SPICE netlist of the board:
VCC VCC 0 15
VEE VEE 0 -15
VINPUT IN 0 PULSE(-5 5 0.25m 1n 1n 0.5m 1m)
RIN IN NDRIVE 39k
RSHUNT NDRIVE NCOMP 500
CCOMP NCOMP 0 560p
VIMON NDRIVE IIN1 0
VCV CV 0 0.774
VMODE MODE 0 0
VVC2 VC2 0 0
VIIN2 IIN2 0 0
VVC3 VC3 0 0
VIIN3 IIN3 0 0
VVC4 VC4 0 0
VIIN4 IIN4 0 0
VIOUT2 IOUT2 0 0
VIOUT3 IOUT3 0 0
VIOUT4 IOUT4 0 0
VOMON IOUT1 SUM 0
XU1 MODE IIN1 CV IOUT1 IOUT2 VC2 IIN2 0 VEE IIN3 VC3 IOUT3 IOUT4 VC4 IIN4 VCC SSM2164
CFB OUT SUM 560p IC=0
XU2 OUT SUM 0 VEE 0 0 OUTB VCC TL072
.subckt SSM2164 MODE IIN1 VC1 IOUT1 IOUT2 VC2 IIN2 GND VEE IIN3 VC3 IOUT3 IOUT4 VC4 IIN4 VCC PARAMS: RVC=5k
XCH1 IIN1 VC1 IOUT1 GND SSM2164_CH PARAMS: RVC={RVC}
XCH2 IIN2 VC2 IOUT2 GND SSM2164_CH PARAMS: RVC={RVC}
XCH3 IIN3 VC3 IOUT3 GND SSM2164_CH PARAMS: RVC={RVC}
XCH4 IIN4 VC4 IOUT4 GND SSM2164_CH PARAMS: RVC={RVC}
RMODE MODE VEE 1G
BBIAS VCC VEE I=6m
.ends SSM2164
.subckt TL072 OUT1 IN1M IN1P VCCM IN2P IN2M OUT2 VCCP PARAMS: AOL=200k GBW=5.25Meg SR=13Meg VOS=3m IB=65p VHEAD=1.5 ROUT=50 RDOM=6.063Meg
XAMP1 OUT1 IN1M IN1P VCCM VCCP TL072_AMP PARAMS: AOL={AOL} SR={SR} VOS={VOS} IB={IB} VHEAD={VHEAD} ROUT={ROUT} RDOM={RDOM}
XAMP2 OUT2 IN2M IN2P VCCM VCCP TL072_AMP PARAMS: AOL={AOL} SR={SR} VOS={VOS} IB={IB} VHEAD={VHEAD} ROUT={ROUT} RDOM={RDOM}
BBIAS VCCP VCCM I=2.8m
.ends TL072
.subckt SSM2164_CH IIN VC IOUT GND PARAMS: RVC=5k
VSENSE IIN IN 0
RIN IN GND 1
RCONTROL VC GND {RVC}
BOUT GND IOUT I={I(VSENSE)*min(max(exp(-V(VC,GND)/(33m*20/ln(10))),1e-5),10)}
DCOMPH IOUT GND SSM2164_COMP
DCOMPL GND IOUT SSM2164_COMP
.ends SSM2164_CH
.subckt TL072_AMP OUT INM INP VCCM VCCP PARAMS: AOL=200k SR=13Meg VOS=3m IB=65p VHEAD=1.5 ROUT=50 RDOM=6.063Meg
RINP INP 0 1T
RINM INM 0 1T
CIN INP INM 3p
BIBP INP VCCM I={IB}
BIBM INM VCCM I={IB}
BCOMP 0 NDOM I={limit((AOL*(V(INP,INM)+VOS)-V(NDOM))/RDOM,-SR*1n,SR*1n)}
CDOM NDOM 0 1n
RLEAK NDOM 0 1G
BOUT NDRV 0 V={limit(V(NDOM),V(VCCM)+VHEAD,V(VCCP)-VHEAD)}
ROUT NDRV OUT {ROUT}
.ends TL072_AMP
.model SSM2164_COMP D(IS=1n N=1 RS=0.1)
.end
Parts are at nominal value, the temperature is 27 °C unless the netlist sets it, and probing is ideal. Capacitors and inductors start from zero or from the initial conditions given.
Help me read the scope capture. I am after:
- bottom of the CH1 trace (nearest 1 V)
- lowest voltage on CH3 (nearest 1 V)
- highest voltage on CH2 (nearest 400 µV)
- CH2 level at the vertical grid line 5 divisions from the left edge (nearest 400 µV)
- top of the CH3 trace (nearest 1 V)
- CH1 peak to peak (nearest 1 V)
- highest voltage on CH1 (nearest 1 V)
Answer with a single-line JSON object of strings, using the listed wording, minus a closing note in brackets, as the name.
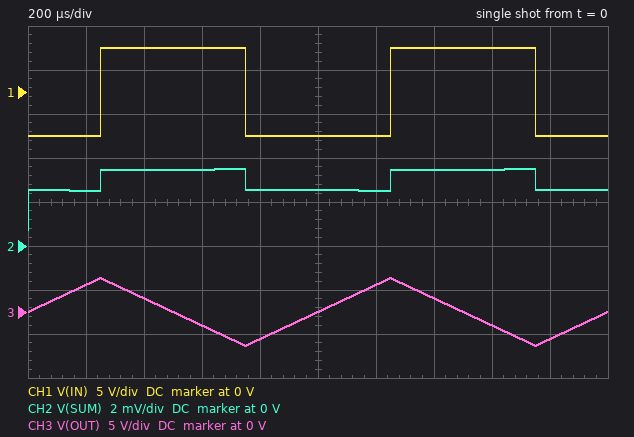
{"bottom of the CH1 trace": "-5 V", "lowest voltage on CH3": "-4 V", "highest voltage on CH2": "3.6 mV", "CH2 level at the vertical grid line 5 divisions from the left edge": "2.4 mV", "top of the CH3 trace": "4 V", "CH1 peak to peak": "10 V", "highest voltage on CH1": "5 V"}
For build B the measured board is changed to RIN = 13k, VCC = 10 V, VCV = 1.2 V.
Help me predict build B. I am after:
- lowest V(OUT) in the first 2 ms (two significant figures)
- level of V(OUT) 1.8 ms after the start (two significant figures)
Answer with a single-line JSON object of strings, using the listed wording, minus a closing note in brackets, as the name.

{"lowest V(OUT) in the first 2 ms": "-2.6 V", "level of V(OUT) 1.8 ms after the start": "-2.1 V"}
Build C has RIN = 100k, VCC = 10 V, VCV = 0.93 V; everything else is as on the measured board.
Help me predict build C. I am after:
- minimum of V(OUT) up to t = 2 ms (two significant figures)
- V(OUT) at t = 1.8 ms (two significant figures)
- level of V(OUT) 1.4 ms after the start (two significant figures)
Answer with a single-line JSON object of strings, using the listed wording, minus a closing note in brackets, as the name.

{"minimum of V(OUT) up to t = 2 ms": "-870 mV", "V(OUT) at t = 1.8 ms": "-690 mV", "level of V(OUT) 1.4 ms after the start": "350 mV"}
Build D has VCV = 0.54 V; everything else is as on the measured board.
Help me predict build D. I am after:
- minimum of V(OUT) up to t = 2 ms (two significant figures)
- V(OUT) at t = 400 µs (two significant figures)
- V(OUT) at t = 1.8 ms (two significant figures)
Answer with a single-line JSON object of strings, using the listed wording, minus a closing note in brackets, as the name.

{"minimum of V(OUT) up to t = 2 ms": "-8.7 V", "V(OUT) at t = 400 µs": "3.5 V", "V(OUT) at t = 1.8 ms": "-7.0 V"}
